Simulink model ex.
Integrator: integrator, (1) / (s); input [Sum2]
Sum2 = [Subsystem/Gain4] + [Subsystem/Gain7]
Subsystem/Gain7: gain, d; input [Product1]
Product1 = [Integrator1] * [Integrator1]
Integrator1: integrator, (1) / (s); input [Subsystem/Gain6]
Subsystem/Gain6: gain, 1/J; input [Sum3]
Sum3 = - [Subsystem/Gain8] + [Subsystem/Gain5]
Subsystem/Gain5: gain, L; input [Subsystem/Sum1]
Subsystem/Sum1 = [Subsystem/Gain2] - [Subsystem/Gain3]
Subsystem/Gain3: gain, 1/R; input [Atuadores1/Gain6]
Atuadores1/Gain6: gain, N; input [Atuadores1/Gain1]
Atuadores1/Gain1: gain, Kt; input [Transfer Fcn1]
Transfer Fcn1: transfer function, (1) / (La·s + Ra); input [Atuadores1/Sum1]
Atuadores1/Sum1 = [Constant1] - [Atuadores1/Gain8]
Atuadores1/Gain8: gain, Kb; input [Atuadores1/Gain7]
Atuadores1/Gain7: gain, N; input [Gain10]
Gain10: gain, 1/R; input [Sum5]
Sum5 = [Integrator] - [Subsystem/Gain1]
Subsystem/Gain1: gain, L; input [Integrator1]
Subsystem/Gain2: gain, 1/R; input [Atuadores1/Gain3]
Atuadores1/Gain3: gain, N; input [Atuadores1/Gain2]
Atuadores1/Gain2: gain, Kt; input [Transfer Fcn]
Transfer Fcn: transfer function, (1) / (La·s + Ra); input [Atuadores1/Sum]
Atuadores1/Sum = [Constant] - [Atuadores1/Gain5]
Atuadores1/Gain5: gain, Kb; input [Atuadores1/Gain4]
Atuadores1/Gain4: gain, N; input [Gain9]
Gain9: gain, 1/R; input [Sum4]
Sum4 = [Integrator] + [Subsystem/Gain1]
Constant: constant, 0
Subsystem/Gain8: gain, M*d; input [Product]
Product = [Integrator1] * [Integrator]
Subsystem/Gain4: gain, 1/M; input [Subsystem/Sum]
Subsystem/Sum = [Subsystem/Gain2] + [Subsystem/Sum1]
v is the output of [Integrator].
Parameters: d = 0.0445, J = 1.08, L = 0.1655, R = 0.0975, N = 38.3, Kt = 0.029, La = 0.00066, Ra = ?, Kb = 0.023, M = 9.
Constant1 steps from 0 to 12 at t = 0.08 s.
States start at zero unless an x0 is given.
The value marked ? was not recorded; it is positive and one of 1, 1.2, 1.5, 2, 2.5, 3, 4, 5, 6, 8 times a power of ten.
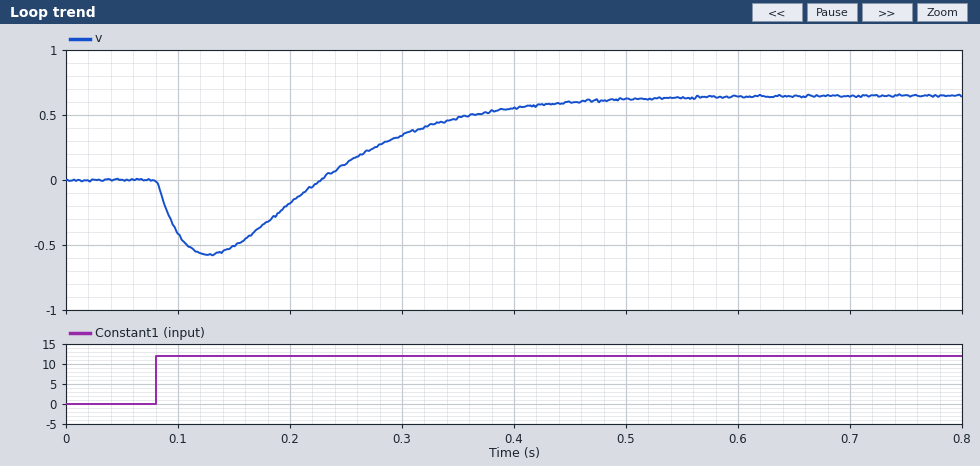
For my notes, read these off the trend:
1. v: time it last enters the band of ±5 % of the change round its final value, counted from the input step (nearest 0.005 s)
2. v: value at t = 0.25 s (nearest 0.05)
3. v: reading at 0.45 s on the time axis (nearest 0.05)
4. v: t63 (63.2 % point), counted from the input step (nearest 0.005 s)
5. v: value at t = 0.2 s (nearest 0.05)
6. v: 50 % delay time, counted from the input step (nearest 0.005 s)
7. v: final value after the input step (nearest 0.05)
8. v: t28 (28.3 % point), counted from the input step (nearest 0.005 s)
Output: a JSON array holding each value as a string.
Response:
["0.410 s", "0.15", "0.60", "0.240 s", "-0.20", "0.215 s", "0.65", "0.180 s"]
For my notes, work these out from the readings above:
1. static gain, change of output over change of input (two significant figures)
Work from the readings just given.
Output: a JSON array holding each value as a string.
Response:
["0.054"]
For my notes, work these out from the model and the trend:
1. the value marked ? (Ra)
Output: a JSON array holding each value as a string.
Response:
["0.5"]
